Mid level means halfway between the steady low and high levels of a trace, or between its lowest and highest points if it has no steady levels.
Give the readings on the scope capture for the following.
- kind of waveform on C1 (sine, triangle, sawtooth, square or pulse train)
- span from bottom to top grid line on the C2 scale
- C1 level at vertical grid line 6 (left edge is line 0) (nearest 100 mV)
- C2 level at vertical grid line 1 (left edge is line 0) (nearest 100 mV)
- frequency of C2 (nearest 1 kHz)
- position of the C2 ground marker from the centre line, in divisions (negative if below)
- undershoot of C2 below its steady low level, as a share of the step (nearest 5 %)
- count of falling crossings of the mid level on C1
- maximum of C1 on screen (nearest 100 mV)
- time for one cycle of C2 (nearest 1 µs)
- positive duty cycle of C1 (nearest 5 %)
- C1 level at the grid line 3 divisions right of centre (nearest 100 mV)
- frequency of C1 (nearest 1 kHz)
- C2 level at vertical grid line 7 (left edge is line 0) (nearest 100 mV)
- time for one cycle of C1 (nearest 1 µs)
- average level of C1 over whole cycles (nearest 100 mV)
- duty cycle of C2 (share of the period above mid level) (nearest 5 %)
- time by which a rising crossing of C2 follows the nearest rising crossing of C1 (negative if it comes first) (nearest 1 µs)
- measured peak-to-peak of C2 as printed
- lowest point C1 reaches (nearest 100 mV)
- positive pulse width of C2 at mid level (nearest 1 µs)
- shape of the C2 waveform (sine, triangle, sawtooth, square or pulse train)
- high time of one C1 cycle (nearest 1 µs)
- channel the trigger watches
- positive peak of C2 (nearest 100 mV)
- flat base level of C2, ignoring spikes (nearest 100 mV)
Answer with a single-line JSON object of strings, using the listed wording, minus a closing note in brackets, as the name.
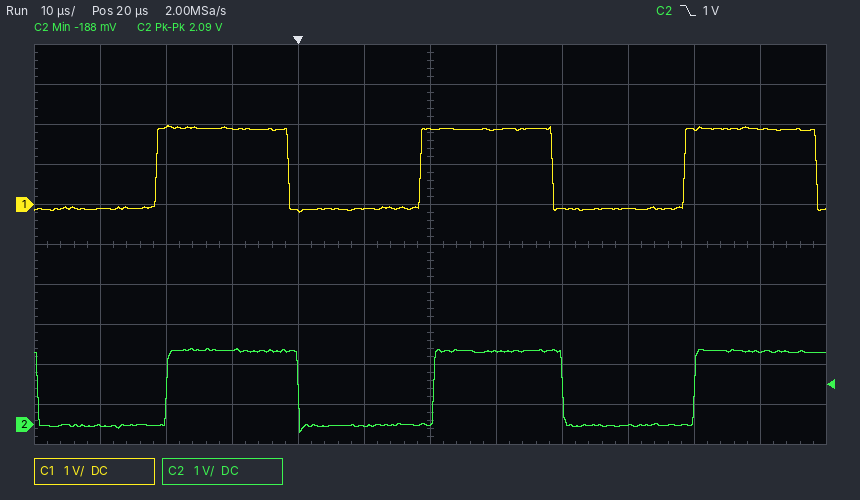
{"kind of waveform on C1": "square", "span from bottom to top grid line on the C2 scale": "10 V", "C1 level at vertical grid line 6 (left edge is line 0)": "1.9 V", "C2 level at vertical grid line 1 (left edge is line 0)": "0.0 V", "frequency of C2": "25 kHz", "position of the C2 ground marker from the centre line, in divisions": "-4.5 div", "undershoot of C2 below its steady low level, as a share of the step": "10 %", "count of falling crossings of the mid level on C1": "3", "maximum of C1 on screen": "2.0 V", "time for one cycle of C2": "40 µs", "positive duty cycle of C1": "50 %", "C1 level at the grid line 3 divisions right of centre": "-100 mV", "frequency of C1": "25 kHz", "C2 level at vertical grid line 7 (left edge is line 0)": "1.8 V", "time for one cycle of C1": "40 µs", "average level of C1 over whole cycles": "900 mV", "duty cycle of C2 (share of the period above mid level)": "50 %", "time by which a rising crossing of C2 follows the nearest rising crossing of C1 (negative if it comes first)": "+2 µs", "measured peak-to-peak of C2 as printed": "2.09 V", "lowest point C1 reaches": "-200 mV", "positive pulse width of C2 at mid level": "20 µs", "shape of the C2 waveform": "square", "high time of one C1 cycle": "20 µs", "channel the trigger watches": "C2", "positive peak of C2": "1.9 V", "flat base level of C2, ignoring spikes": "0.0 V"}
